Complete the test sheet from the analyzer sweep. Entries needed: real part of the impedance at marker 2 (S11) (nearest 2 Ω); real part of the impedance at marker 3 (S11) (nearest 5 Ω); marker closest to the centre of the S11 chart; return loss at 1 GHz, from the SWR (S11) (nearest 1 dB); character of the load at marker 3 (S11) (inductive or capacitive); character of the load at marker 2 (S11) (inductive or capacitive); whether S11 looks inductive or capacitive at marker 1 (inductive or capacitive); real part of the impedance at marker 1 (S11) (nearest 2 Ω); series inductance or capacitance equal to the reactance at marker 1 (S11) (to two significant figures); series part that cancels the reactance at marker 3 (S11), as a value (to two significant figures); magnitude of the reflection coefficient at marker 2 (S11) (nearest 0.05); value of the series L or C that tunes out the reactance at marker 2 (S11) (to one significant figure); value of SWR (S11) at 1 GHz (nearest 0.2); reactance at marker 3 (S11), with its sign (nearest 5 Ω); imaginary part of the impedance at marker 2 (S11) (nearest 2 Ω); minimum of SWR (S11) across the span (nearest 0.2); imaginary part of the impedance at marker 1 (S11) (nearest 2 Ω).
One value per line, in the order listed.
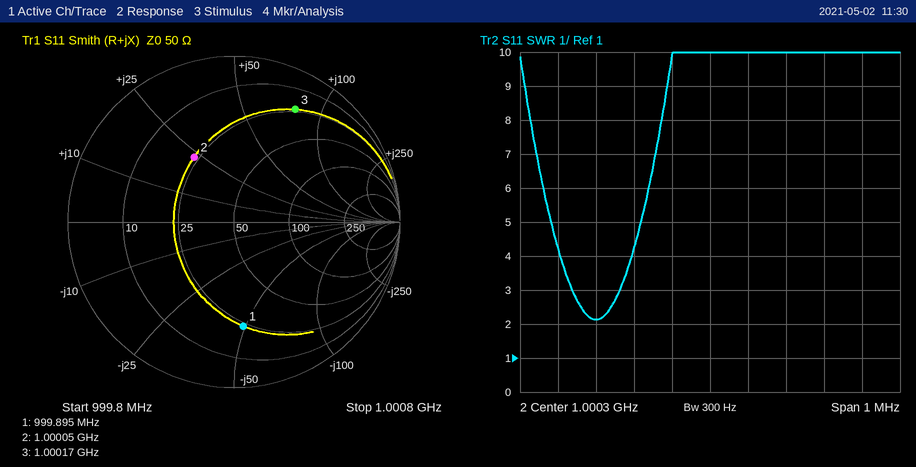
24 Ω
25 Ω
marker 2
9 dB
inductive
inductive
capacitive
24 Ω
3.3 pF
2.0 pF
0.45
7 pF
2.2
+80 Ω
+24 Ω
2.2
-48 Ω
